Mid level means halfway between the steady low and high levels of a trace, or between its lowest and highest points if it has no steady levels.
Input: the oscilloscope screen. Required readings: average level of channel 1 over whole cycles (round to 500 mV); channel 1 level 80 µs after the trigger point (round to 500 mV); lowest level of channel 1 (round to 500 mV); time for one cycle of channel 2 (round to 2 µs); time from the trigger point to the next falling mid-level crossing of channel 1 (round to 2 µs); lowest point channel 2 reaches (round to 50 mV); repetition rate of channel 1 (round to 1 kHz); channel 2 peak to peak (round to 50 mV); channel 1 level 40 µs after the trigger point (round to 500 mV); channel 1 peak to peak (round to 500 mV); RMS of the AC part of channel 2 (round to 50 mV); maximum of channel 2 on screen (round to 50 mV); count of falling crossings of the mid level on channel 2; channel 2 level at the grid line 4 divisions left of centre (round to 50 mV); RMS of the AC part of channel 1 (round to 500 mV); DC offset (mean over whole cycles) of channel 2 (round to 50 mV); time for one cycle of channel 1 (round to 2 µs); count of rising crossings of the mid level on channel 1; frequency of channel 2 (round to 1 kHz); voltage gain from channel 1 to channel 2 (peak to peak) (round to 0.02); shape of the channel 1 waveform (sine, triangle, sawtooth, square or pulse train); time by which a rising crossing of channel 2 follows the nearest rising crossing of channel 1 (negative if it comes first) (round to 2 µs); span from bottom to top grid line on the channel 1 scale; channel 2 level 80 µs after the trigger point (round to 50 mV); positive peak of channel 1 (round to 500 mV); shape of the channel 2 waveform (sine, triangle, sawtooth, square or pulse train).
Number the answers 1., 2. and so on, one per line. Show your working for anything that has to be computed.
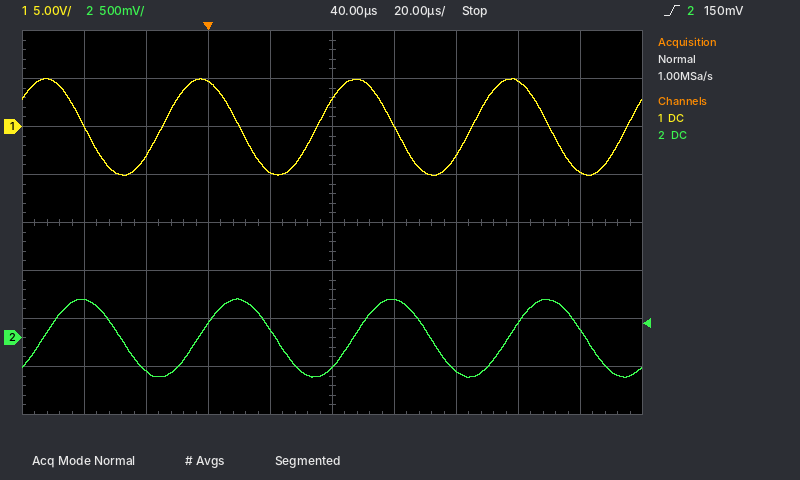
1. (5.0 V + (-5.0 V)) / 2 ≈ 0.0 V
2. -3.0 V
3. -5.0 V
4. 50 µs
5. 10 µs
6. -400 mV
7. 1 / 50 µs ≈ 20 kHz
8. 400 mV − (-400 mV) = 800 mV
9. 3.0 V
10. 5.0 V − (-5.0 V) = 10.0 V
11. 800 mV / (2√2) ≈ 283 mV, so 300 mV to the nearest 50 mV
12. 400 mV
13. 4
14. 400 mV
15. 10.0 V / (2√2) ≈ 3.5 V
16. (400 mV + (-400 mV)) / 2 ≈ 0 mV
17. 50 µs
18. 4
19. 1 / 50 µs ≈ 20 kHz
20. 800 mV / 10.0 V ≈ 0.08
21. sine
22. +12 µs
23. 40 V
24. -350 mV
25. 5.0 V
26. sine
